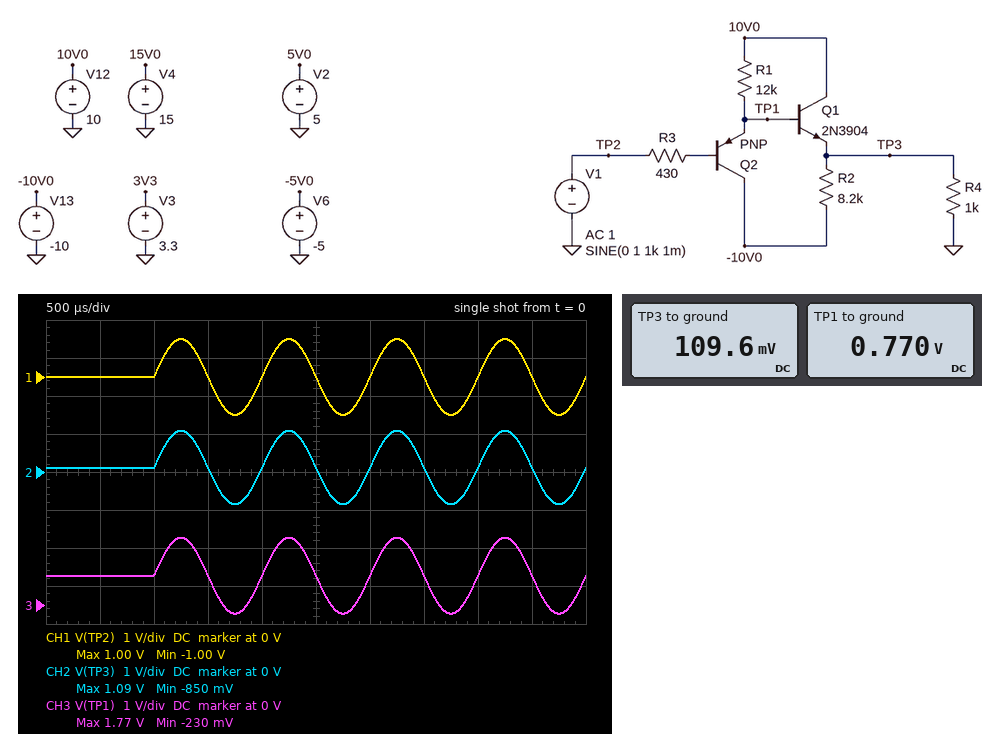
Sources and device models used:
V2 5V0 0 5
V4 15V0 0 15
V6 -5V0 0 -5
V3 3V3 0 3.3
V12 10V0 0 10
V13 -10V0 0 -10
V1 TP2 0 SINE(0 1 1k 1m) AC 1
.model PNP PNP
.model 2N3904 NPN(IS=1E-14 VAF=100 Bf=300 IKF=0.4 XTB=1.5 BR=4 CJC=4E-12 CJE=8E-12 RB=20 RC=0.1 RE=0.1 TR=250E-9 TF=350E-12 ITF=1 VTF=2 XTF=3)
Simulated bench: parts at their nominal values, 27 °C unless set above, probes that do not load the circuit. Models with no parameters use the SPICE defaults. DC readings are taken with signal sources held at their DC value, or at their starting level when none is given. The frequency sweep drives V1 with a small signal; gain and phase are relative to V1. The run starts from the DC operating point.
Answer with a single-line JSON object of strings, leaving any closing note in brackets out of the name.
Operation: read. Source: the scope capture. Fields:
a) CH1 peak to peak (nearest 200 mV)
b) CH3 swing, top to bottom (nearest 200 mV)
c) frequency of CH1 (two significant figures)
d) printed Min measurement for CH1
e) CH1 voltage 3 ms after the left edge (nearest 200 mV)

{"CH1 peak to peak": "2.0 V", "CH3 swing, top to bottom": "2.0 V", "frequency of CH1": "1.0 kHz", "printed Min measurement for CH1": "-1.00 V", "CH1 voltage 3 ms after the left edge": "0 V"}
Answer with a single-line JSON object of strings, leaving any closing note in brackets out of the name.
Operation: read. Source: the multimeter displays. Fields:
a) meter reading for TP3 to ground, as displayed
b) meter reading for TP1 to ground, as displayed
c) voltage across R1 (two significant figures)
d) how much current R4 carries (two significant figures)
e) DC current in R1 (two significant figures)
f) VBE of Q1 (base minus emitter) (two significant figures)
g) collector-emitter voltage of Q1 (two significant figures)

{"meter reading for TP3 to ground, as displayed": "109.6 mV", "meter reading for TP1 to ground, as displayed": "0.770 V", "voltage across R1": "9.2 V", "how much current R4 carries": "110 µA", "DC current in R1": "770 µA", "VBE of Q1 (base minus emitter)": "660 mV", "collector-emitter voltage of Q1": "9.9 V"}
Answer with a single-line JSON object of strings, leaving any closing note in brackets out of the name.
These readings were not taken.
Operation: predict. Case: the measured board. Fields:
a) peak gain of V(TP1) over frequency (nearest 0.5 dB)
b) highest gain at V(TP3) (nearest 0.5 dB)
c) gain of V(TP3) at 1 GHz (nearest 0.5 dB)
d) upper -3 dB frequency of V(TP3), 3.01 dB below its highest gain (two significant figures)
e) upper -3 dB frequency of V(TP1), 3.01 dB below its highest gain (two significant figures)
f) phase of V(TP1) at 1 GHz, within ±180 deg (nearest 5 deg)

{"peak gain of V(TP1) over frequency": "0 dB", "highest gain at V(TP3)": "0 dB", "gain of V(TP3) at 1 GHz": "-2.0 dB", "upper -3 dB frequency of V(TP3), 3.01 dB below its highest gain": "1.6 GHz", "upper -3 dB frequency of V(TP1), 3.01 dB below its highest gain": "1.8 GHz", "phase of V(TP1) at 1 GHz, within ±180 deg": "-20 deg"}
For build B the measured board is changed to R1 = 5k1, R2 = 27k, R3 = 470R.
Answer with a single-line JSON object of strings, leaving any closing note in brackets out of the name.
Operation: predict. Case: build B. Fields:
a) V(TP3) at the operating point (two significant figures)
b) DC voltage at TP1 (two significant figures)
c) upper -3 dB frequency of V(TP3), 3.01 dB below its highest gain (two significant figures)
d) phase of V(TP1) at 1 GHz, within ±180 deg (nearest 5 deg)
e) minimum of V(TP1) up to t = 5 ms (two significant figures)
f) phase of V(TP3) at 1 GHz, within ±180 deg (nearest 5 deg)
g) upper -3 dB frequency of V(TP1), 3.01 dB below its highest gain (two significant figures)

{"V(TP3) at the operating point": "160 mV", "DC voltage at TP1": "800 mV", "upper -3 dB frequency of V(TP3), 3.01 dB below its highest gain": "2.5 GHz", "phase of V(TP1) at 1 GHz, within ±180 deg": "-10 deg", "minimum of V(TP1) up to t = 5 ms": "-200 mV", "phase of V(TP3) at 1 GHz, within ±180 deg": "-20 deg", "upper -3 dB frequency of V(TP1), 3.01 dB below its highest gain": "3.5 GHz"}
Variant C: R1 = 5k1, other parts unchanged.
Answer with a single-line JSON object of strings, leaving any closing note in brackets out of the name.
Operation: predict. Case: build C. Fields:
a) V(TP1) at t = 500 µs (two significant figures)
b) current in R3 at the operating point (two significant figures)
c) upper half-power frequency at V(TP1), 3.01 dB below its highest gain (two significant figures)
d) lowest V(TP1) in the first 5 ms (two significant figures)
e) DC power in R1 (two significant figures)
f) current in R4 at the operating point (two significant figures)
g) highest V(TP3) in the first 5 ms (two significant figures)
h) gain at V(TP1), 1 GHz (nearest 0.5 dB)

{"V(TP1) at t = 500 µs": "800 mV", "current in R3 at the operating point": "18 µA", "upper half-power frequency at V(TP1), 3.01 dB below its highest gain": "3.6 GHz", "lowest V(TP1) in the first 5 ms": "-200 mV", "DC power in R1": "17 mW", "current in R4 at the operating point": "140 µA", "highest V(TP3) in the first 5 ms": "1.1 V", "gain at V(TP1), 1 GHz": "-0.5 dB"}
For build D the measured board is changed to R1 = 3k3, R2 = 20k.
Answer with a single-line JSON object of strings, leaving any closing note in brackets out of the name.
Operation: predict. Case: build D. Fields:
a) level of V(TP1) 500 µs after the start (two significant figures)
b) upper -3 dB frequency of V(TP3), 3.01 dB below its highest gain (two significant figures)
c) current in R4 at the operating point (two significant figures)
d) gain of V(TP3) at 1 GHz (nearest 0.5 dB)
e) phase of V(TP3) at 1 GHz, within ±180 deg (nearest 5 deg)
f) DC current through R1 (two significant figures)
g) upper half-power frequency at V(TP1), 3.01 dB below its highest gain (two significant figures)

{"level of V(TP1) 500 µs after the start": "810 mV", "upper -3 dB frequency of V(TP3), 3.01 dB below its highest gain": "2.9 GHz", "current in R4 at the operating point": "170 µA", "gain of V(TP3) at 1 GHz": "-1.0 dB", "phase of V(TP3) at 1 GHz, within ±180 deg": "-20 deg", "DC current through R1": "2.8 mA", "upper half-power frequency at V(TP1), 3.01 dB below its highest gain": "5.2 GHz"}
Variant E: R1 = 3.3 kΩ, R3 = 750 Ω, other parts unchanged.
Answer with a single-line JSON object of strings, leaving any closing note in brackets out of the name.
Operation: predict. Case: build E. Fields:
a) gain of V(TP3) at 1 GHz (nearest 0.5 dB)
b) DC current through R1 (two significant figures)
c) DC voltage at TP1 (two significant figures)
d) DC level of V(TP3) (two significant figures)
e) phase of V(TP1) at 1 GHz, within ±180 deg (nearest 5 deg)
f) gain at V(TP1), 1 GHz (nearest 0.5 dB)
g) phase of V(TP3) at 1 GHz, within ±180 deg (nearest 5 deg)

{"gain of V(TP3) at 1 GHz": "-1.0 dB", "DC current through R1": "2.8 mA", "DC voltage at TP1": "820 mV", "DC level of V(TP3)": "160 mV", "phase of V(TP1) at 1 GHz, within ±180 deg": "-10 deg", "gain at V(TP1), 1 GHz": "-0.5 dB", "phase of V(TP3) at 1 GHz, within ±180 deg": "-20 deg"}
